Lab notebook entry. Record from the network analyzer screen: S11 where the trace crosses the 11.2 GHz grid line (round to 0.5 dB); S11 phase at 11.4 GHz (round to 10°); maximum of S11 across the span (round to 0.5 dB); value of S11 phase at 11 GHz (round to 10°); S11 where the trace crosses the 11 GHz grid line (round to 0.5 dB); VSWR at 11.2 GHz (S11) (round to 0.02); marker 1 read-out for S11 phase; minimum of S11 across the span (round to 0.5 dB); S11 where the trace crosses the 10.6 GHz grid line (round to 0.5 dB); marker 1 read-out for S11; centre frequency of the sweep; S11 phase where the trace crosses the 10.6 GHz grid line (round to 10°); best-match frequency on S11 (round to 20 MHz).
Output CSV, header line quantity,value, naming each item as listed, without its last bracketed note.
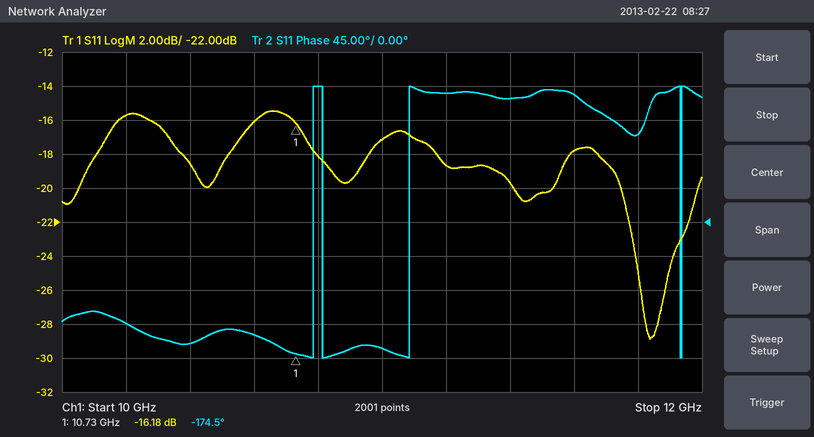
quantity,value
S11 where the trace crosses the 11.2 GHz grid line,-18.5 dB
S11 phase at 11.4 GHz,160°
maximum of S11 across the span,-15.5 dB
value of S11 phase at 11 GHz,-170°
S11 where the trace crosses the 11 GHz grid line,-17.0 dB
VSWR at 11.2 GHz (S11),1.26
marker 1 read-out for S11 phase,-174.5°
minimum of S11 across the span,-29.0 dB
S11 where the trace crosses the 10.6 GHz grid line,-16.0 dB
marker 1 read-out for S11,-16.18 dB
centre frequency of the sweep,11 GHz
S11 phase where the trace crosses the 10.6 GHz grid line,-150°
best-match frequency on S11,11.84 GHz
